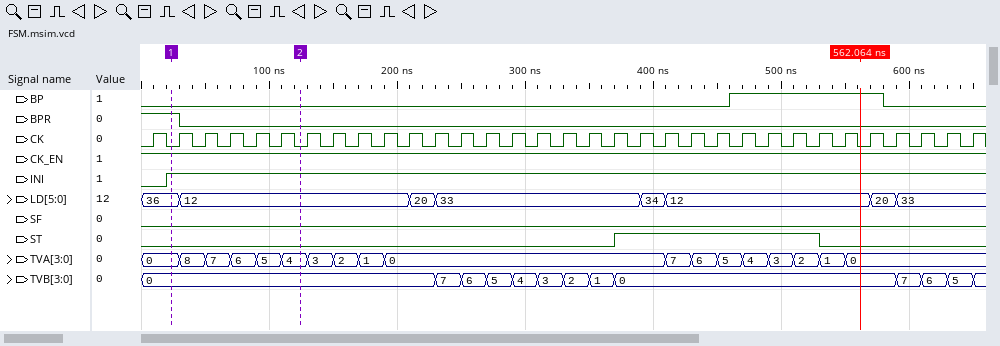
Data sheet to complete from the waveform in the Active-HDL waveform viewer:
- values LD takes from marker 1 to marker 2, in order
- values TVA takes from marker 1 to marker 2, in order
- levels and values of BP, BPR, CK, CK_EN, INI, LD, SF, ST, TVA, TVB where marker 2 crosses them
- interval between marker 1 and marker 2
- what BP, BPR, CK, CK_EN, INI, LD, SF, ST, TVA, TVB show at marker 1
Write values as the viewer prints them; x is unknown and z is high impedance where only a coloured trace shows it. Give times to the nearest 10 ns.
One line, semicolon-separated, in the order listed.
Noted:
36, 12; 0, 8, 7, 6, 5, 4; BP=0, BPR=0, CK=0, CK_EN=1, INI=1, LD=12, SF=0, ST=0, TVA=4, TVB=0; 100 ns; BP=0, BPR=1, CK=0, CK_EN=1, INI=1, LD=36, SF=0, ST=0, TVA=0, TVB=0
